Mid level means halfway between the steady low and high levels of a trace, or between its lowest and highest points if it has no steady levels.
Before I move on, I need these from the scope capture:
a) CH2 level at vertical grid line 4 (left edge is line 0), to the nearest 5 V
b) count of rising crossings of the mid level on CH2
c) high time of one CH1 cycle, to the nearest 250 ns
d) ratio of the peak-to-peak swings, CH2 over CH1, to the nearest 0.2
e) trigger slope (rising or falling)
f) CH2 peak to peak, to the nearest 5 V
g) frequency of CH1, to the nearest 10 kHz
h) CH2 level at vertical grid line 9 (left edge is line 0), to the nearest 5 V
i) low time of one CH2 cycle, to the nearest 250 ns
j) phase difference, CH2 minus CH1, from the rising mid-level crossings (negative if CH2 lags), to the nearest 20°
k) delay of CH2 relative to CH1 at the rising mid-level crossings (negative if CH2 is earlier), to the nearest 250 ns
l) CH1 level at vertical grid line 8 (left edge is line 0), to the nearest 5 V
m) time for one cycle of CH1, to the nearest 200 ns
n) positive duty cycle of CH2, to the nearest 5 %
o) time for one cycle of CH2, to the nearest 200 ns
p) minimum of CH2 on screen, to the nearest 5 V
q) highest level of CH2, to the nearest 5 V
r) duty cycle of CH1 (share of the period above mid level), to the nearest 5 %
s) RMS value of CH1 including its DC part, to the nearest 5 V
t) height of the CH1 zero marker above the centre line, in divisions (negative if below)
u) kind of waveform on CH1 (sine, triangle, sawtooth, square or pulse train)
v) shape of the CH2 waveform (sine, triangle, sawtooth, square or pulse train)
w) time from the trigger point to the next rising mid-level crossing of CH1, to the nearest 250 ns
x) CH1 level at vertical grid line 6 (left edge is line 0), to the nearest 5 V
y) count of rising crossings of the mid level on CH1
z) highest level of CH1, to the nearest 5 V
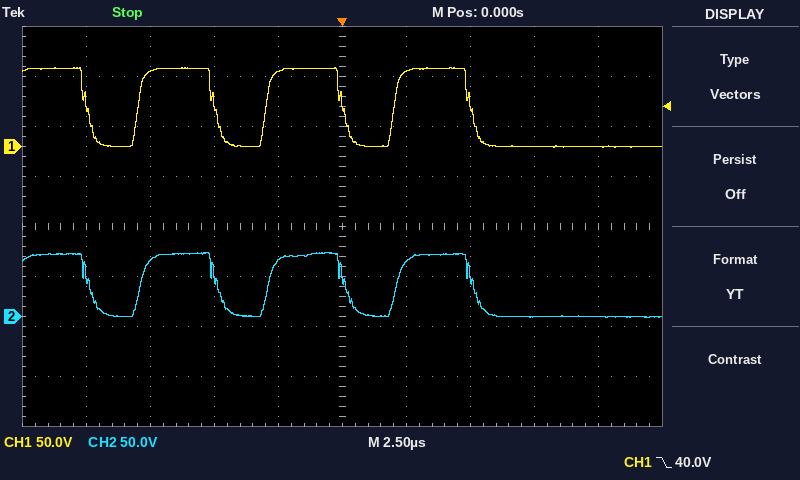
55 V
3
3.00 µs
0.8
falling
65 V
200 kHz
0 V
2.00 µs
0°
0.00 µs
0 V
5.0 µs
60 %
5.0 µs
0 V
65 V
60 %
60 V
+1.6 div
pulse train
pulse train
2.00 µs
75 V
3
80 V
